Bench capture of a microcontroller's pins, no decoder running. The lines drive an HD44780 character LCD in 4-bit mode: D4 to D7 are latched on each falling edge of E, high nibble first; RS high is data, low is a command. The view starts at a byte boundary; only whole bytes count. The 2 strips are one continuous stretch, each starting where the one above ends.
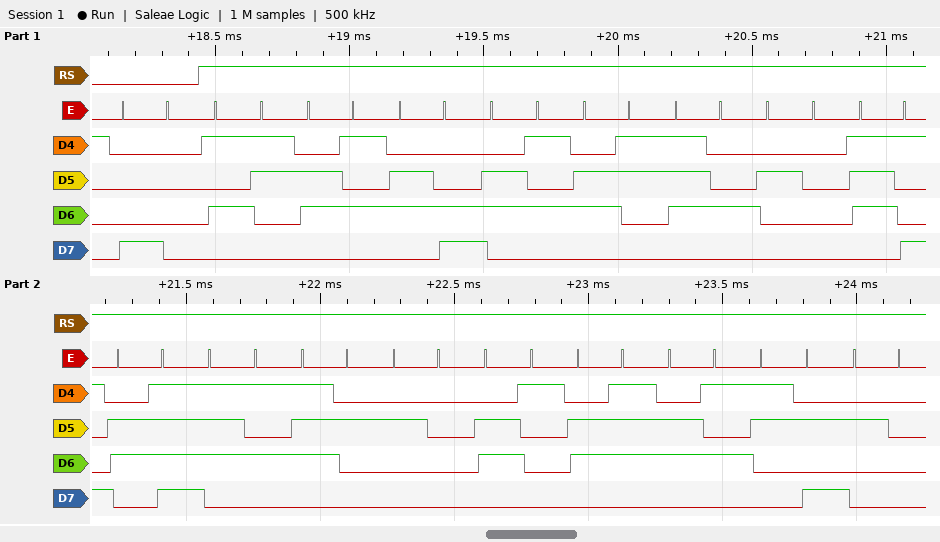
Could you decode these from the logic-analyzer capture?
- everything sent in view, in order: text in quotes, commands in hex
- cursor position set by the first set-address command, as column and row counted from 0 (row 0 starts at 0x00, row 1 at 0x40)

0x80 "Select your age: "
column 0, row 0
